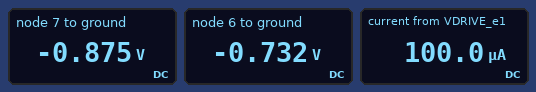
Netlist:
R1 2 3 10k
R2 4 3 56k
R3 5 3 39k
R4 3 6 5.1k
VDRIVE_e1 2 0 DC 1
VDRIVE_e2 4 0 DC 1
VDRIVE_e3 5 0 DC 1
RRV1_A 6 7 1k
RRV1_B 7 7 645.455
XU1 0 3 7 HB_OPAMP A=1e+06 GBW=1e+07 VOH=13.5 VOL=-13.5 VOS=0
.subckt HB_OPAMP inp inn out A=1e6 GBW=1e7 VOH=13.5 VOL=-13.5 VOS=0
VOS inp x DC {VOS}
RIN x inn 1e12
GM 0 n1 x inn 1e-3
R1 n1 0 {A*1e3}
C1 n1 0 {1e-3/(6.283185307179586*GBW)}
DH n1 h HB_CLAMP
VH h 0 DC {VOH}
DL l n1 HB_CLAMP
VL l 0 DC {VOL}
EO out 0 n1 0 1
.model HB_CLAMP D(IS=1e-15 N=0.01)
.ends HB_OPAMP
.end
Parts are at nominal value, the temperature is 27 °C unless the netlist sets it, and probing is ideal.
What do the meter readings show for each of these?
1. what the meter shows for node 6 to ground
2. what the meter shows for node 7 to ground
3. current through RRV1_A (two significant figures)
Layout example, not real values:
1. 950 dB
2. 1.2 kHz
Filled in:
1. -0.732 V
2. -0.875 V
3. 140 µA
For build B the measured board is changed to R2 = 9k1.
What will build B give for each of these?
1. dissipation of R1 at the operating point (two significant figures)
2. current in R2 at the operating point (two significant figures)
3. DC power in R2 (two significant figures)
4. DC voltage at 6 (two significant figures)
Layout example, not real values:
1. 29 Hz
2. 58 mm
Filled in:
1. 100 µW
2. 110 µA
3. 110 µW
4. -1.2 V
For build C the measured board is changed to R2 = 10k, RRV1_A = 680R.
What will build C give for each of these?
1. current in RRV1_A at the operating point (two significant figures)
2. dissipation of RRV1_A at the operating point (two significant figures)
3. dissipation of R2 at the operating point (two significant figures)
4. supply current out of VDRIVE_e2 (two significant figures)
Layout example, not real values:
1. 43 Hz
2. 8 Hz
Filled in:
1. 230 µA
2. 35 µW
3. 100 µW
4. 100 µA
